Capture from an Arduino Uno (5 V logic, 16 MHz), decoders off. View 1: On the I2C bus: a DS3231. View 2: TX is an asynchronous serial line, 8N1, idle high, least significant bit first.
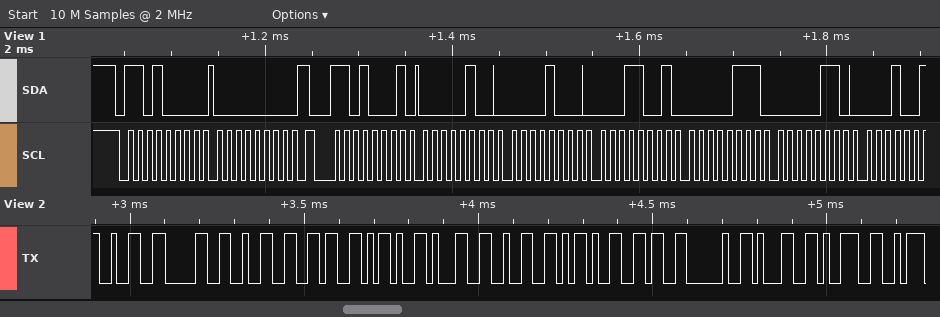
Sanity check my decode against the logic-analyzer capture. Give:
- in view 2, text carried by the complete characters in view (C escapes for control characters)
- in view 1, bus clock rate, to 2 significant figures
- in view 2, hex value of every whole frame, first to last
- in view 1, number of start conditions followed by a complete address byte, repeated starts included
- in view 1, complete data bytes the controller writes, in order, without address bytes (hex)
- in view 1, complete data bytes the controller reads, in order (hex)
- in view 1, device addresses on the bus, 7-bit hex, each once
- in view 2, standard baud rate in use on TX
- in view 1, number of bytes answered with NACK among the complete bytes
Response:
"2026-12-6 19"
100 kHz
32 30 32 36 2D 31 32 2D 36 20 31 39
2
00
04 08 19 07 06
0x68
57600 baud
0
